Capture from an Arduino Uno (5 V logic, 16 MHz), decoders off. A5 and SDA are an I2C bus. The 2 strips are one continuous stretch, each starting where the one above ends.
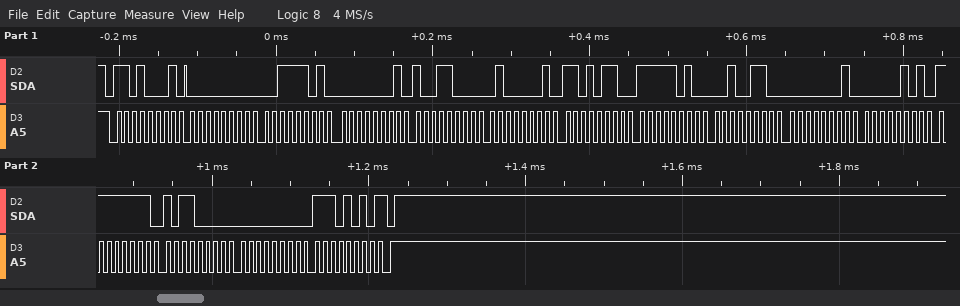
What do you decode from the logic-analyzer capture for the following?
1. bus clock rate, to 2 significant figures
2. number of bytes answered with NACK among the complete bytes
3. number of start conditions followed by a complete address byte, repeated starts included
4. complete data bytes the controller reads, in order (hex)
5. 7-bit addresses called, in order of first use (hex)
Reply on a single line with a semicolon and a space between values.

100 kHz; 1; 1; 00 3D 01 98 41 D6 FA 26 01 05 FF B0 00 EA; 0x68
